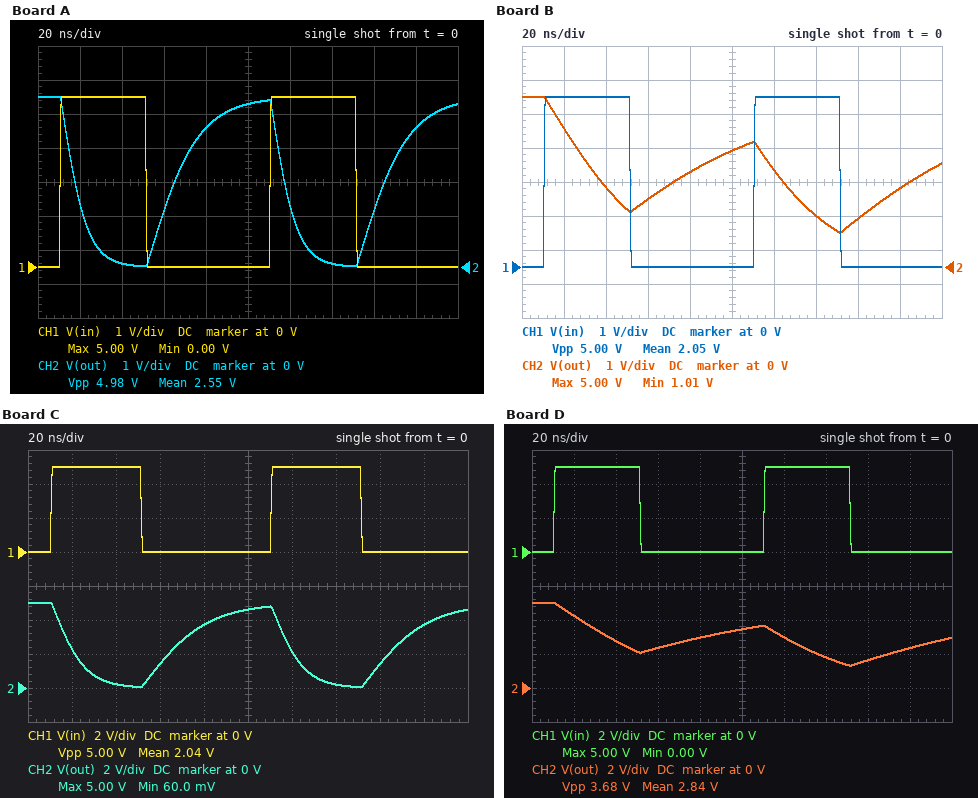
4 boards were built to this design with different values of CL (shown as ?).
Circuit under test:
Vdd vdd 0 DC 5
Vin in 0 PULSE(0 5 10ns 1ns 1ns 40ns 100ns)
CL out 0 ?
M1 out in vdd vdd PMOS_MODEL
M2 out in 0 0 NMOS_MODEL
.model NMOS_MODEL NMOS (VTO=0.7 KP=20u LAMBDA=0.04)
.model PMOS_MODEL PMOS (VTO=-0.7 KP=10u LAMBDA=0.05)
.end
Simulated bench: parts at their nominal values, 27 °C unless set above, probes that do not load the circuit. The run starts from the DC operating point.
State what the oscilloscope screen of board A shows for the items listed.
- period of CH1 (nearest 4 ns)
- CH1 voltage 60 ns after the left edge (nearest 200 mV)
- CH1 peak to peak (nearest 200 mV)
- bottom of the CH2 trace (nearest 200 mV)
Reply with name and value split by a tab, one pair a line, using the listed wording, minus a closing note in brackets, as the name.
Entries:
period of CH1	100 ns
CH1 voltage 60 ns after the left edge	0 V
CH1 peak to peak	5.0 V
bottom of the CH2 trace	0 V
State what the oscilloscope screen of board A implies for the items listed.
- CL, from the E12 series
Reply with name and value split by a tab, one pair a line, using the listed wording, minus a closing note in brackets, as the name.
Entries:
CL, from the E12 series	560 fF
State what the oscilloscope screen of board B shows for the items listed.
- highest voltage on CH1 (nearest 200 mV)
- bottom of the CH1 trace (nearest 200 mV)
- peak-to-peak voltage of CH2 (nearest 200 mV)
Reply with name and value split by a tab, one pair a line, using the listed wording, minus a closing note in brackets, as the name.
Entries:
highest voltage on CH1	5.0 V
bottom of the CH1 trace	0 V
peak-to-peak voltage of CH2	4.0 V
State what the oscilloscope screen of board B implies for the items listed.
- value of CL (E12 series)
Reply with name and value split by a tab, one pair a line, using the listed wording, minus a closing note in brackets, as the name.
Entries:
value of CL	2.2 pF
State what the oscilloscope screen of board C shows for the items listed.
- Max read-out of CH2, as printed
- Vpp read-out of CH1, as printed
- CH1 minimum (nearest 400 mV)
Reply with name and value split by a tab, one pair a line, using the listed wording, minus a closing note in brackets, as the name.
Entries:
Max read-out of CH2, as printed	5.00 V
Vpp read-out of CH1, as printed	5.00 V
CH1 minimum	0 V
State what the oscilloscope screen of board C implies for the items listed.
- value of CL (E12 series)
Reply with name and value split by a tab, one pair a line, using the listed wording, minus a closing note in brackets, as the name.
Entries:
value of CL	680 fF
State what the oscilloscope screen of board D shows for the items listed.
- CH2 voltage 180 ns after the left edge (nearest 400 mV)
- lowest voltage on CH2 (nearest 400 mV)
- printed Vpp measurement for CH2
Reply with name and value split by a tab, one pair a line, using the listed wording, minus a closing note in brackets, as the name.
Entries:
CH2 voltage 180 ns after the left edge	2.4 V
lowest voltage on CH2	1.2 V
printed Vpp measurement for CH2	3.68 V
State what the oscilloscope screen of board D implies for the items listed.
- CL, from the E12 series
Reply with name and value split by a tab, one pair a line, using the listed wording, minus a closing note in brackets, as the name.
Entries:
CL, from the E12 series	2.7 pF
